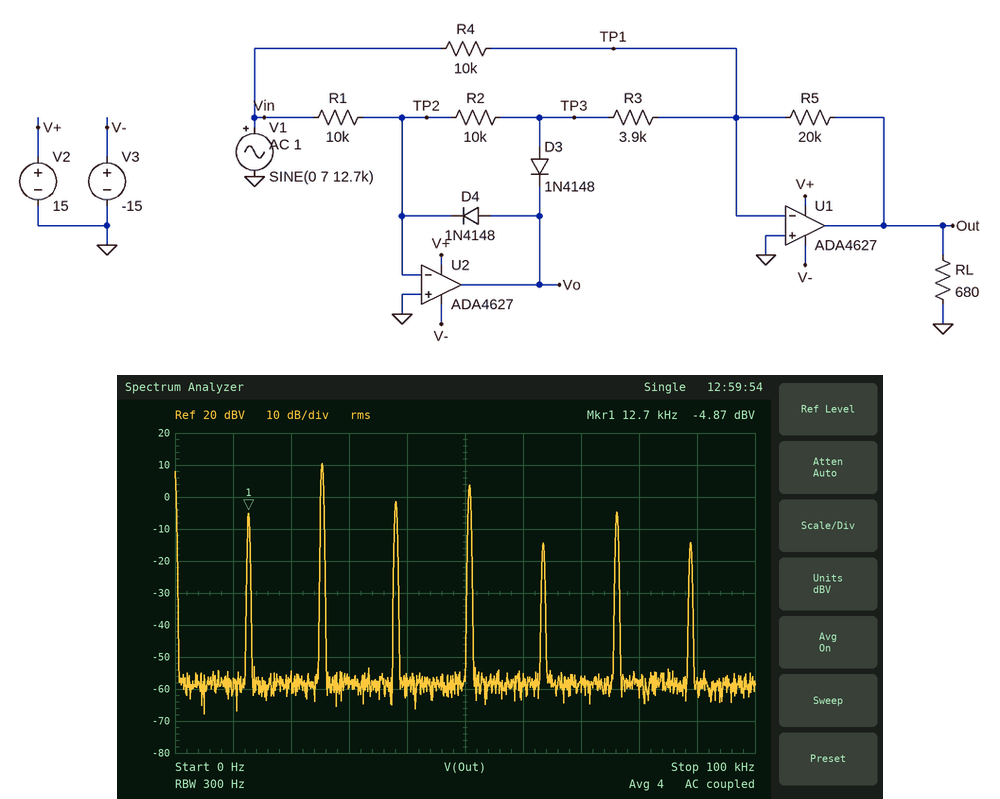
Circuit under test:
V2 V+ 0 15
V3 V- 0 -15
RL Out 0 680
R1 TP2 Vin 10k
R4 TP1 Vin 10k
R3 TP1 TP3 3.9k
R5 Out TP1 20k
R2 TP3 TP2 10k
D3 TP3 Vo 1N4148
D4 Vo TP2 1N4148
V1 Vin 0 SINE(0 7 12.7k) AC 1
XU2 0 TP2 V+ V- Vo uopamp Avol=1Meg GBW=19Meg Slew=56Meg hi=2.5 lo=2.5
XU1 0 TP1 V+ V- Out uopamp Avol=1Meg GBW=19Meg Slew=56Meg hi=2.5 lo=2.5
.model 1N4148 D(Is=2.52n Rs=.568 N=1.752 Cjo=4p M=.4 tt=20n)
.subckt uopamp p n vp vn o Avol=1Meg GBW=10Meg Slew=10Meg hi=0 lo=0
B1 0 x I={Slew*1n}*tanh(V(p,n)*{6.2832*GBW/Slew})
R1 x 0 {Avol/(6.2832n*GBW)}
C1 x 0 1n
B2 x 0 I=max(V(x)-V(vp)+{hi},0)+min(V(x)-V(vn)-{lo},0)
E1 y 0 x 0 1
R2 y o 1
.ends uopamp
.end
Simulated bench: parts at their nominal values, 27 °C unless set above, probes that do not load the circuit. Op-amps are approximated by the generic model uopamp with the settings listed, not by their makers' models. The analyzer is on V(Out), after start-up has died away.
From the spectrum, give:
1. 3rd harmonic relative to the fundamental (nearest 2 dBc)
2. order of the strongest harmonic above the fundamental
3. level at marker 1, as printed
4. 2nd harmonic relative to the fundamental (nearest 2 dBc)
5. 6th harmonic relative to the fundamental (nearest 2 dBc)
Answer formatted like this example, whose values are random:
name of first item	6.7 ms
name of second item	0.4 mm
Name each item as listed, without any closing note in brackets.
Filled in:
3rd harmonic relative to the fundamental	4 dBc
order of the strongest harmonic above the fundamental	2
level at marker 1, as printed	-4.87 dBV
2nd harmonic relative to the fundamental	16 dBc
6th harmonic relative to the fundamental	0 dBc
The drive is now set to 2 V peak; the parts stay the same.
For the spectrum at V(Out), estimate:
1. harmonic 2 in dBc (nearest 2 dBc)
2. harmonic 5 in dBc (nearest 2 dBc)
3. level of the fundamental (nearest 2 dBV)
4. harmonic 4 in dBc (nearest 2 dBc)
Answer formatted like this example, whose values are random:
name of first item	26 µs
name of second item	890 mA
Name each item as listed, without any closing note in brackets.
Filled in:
harmonic 2 in dBc	6 dBc
harmonic 5 in dBc	-46 dBc
level of the fundamental	-2 dBV
harmonic 4 in dBc	-8 dBc
